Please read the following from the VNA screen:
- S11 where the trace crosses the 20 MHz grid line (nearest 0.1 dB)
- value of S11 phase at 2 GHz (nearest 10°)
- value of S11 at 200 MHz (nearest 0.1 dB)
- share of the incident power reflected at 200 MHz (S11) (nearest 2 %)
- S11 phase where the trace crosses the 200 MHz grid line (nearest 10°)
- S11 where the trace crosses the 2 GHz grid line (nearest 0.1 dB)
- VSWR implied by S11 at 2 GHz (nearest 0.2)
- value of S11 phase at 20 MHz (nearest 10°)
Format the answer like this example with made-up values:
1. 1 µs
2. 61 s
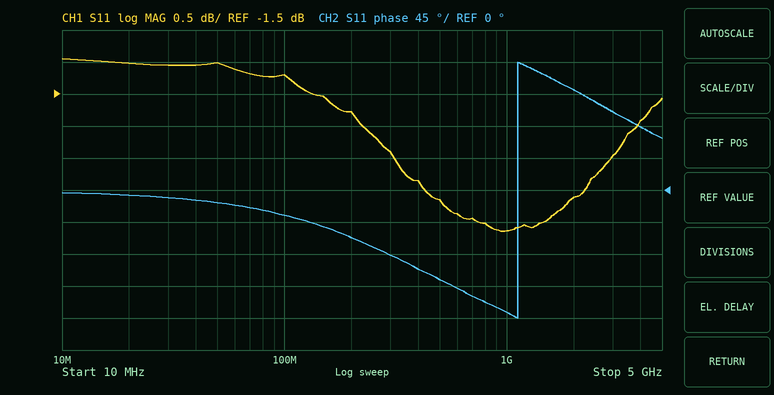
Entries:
1. -1.0 dB
2. 140°
3. -1.8 dB
4. 66 %
5. -70°
6. -3.1 dB
7. 5.6
8. -10°
